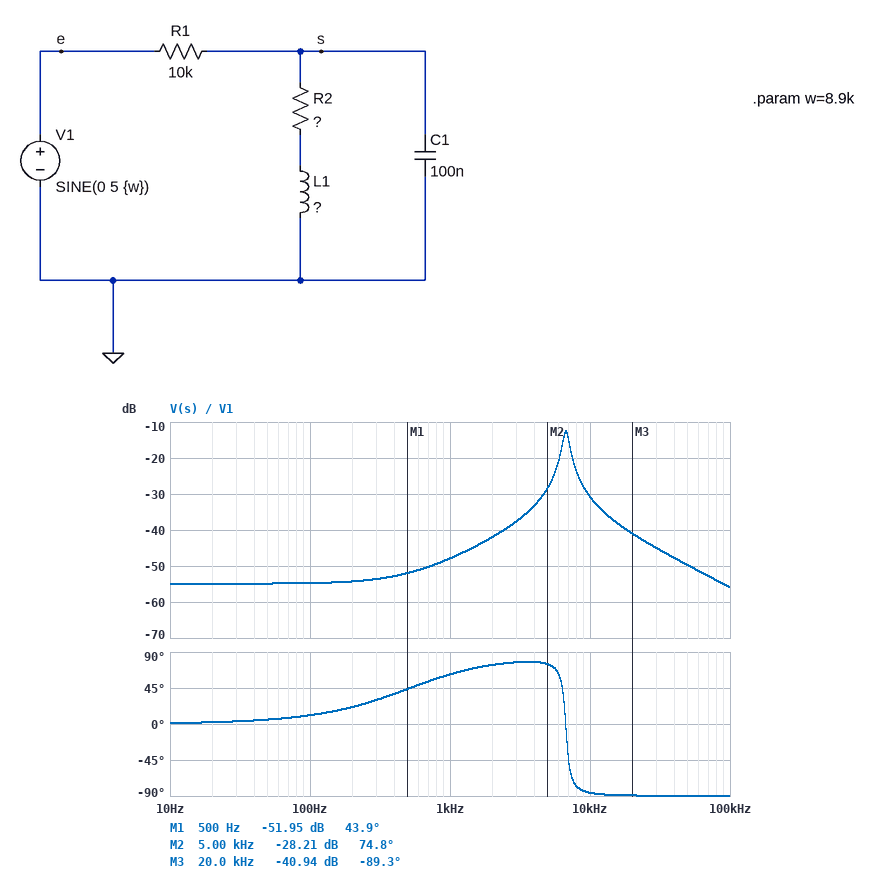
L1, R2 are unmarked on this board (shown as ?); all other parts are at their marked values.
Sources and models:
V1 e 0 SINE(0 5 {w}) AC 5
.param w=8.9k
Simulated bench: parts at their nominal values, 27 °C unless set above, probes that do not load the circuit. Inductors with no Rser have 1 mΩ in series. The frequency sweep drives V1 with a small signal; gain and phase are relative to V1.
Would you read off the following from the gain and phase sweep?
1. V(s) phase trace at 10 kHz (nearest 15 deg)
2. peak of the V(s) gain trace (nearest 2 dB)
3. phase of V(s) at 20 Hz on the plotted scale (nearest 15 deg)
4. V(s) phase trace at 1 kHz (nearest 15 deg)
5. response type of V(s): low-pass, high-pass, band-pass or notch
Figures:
-90 deg
-12 dB
0 deg
60 deg
band-pass
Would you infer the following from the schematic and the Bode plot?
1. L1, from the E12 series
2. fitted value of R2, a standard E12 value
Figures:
5.6 mH
18 Ω
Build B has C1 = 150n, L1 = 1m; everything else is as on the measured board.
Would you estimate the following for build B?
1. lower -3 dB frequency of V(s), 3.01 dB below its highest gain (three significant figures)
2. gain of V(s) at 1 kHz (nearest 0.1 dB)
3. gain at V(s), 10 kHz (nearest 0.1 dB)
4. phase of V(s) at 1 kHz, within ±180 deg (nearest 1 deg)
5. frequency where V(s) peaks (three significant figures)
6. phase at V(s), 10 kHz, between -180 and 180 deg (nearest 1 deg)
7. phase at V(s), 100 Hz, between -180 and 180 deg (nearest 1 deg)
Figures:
11.6 kHz
-54.4 dB
-36.7 dB
18 deg
13.0 kHz
51 deg
2 deg
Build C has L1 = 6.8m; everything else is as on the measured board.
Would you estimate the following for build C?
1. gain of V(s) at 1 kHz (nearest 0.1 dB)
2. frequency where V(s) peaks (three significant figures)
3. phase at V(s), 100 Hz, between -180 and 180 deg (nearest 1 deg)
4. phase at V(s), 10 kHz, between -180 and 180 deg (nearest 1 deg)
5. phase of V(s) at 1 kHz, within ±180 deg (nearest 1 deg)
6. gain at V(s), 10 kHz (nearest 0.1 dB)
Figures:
-46.5 dB
6.11 kHz
13 deg
-87 deg
66 deg
-31.9 dB
